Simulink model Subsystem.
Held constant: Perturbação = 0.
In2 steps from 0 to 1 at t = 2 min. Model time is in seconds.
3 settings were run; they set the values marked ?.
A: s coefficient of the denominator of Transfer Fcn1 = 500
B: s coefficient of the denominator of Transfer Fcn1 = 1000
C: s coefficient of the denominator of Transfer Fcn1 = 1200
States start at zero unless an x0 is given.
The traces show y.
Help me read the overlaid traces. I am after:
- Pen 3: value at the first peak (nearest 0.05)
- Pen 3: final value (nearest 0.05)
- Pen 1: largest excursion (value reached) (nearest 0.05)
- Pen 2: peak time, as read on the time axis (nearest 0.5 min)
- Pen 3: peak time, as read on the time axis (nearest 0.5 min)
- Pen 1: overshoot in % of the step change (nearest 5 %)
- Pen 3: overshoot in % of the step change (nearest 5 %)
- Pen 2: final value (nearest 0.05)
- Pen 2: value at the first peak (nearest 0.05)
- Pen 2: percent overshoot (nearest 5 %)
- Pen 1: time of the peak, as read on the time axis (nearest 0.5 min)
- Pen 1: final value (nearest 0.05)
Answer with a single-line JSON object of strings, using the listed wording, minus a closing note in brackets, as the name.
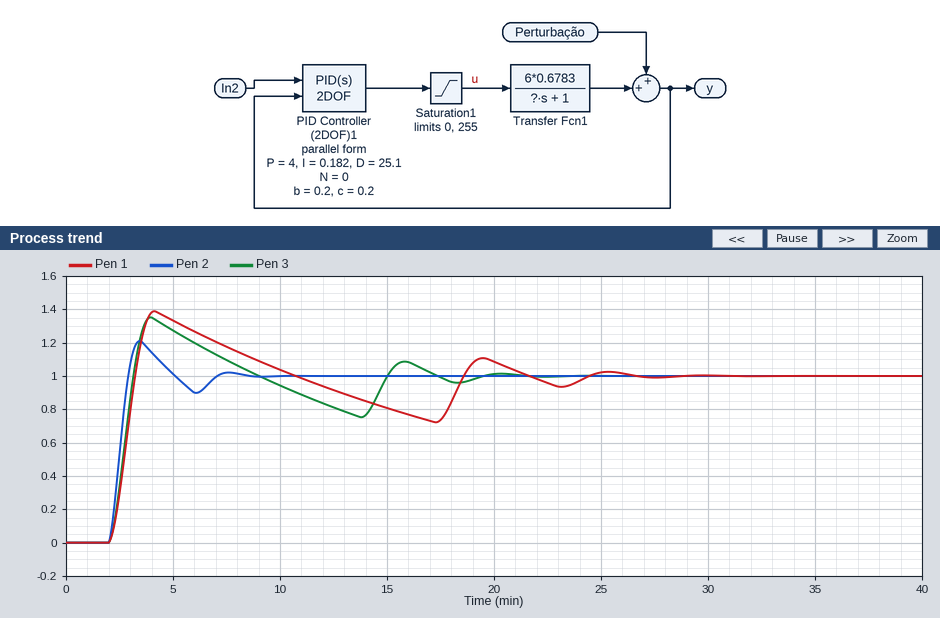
{"Pen 3: value at the first peak": "1.35", "Pen 3: final value": "1.00", "Pen 1: largest excursion (value reached)": "1.40", "Pen 2: peak time, as read on the time axis": "3.5 min", "Pen 3: peak time, as read on the time axis": "4.0 min", "Pen 1: overshoot in % of the step change": "40 %", "Pen 3: overshoot in % of the step change": "35 %", "Pen 2: final value": "1.00", "Pen 2: value at the first peak": "1.20", "Pen 2: percent overshoot": "20 %", "Pen 1: time of the peak, as read on the time axis": "4.0 min", "Pen 1: final value": "1.00"}
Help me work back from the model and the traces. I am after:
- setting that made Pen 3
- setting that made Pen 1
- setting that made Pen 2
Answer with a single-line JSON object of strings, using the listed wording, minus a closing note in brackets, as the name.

{"setting that made Pen 3": "B", "setting that made Pen 1": "C", "setting that made Pen 2": "A"}
